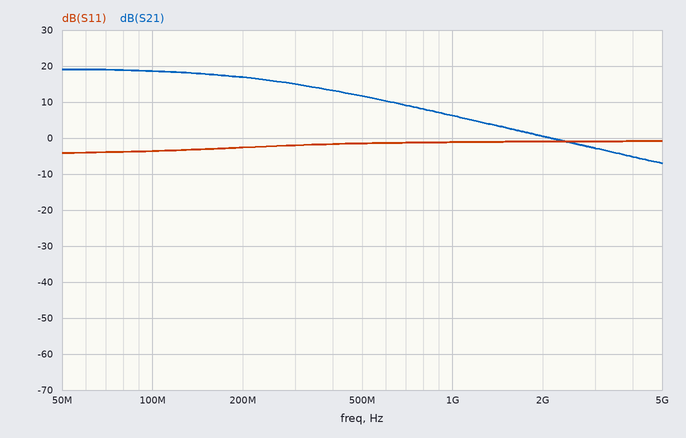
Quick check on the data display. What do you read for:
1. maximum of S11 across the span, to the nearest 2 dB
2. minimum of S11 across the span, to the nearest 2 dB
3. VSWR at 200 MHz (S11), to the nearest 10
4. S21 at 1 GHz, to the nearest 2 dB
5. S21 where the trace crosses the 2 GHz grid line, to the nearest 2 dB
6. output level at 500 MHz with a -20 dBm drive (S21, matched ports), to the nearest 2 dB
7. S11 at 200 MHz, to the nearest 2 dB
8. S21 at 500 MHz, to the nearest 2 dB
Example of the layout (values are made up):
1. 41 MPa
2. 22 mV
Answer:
1. 0 dB
2. -4 dB
3. 10
4. 6 dB
5. 0 dB
6. -8 dBm
7. -2 dB
8. 12 dB
